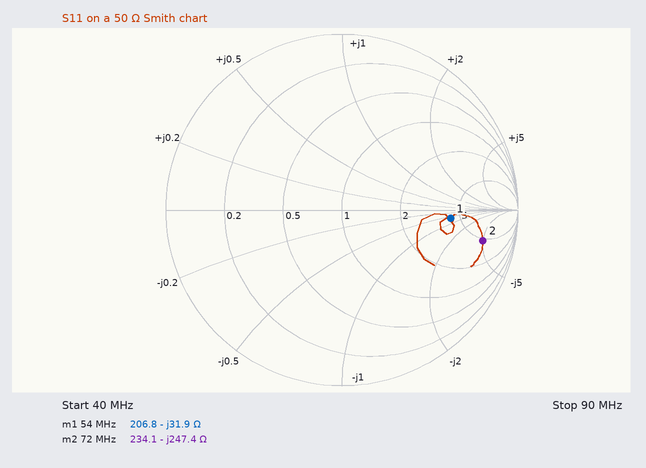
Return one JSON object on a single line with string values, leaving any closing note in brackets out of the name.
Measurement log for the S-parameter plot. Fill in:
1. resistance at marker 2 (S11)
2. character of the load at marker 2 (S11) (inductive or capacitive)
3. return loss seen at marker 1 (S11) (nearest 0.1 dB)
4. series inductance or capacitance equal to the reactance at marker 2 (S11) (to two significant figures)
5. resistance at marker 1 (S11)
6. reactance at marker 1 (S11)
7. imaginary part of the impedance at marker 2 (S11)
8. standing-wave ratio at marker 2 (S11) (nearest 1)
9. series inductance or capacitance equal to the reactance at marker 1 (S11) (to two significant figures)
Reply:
{"resistance at marker 2": "234.1 Ω", "character of the load at marker 2 (S11)": "capacitive", "return loss seen at marker 1 (S11)": "4.2 dB", "series inductance or capacitance equal to the reactance at marker 2 (S11)": "8.9 pF", "resistance at marker 1": "206.8 Ω", "reactance at marker 1": "-31.9 Ω", "imaginary part of the impedance at marker 2": "-247.4 Ω", "standing-wave ratio at marker 2 (S11)": "10", "series inductance or capacitance equal to the reactance at marker 1 (S11)": "92 pF"}
